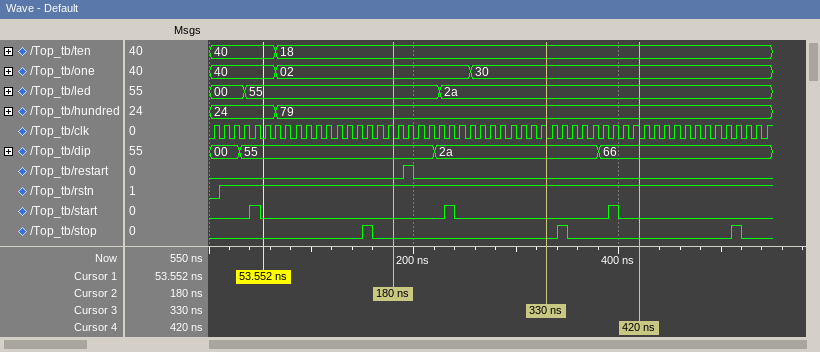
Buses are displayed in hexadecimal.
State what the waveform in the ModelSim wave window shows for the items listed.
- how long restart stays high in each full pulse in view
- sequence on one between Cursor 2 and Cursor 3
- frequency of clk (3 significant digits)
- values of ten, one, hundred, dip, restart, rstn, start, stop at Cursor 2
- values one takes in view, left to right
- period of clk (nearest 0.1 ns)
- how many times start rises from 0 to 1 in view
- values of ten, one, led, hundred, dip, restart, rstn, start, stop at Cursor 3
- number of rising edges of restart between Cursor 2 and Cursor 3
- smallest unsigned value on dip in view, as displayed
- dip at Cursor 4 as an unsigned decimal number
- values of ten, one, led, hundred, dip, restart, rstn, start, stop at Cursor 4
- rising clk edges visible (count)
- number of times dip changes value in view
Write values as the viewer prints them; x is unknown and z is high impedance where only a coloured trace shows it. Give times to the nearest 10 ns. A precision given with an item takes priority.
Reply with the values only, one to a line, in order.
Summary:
10 ns
02, 30
100 MHz
ten=18, one=02, hundred=79, dip=55, restart=0, rstn=1, start=0, stop=0
40, 02, 30
10 ns
3
ten=18, one=30, led=2a, hundred=79, dip=2a, restart=0, rstn=1, start=0, stop=0
1
00
102
ten=18, one=30, led=2a, hundred=79, dip=66, restart=0, rstn=1, start=0, stop=0
55
3
